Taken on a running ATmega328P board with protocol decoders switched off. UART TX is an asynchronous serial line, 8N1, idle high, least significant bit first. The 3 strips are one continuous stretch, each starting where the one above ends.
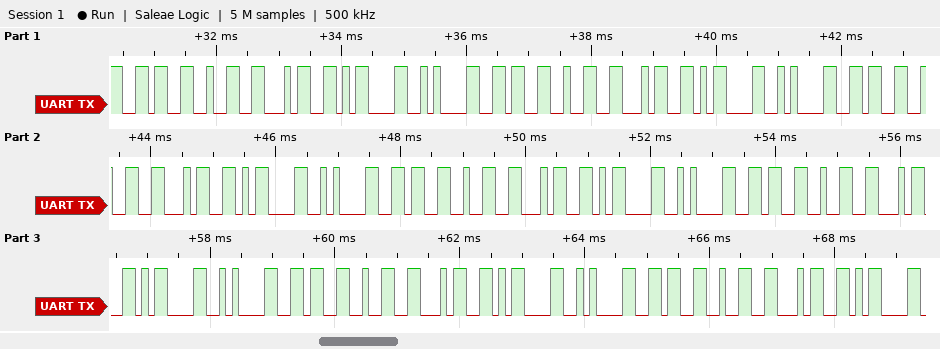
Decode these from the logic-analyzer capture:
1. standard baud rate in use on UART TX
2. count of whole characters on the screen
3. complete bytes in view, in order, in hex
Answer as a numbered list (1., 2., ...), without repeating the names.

1. 9600 baud
2. 34
3. 36 32 34 0D 0A 36 32 34 0D 0A 36 32 34 0D 0A 36 32 34 0D 0A 36 32 34 0D 0A 36 32 34 0D 0A 36 32 34 0D
